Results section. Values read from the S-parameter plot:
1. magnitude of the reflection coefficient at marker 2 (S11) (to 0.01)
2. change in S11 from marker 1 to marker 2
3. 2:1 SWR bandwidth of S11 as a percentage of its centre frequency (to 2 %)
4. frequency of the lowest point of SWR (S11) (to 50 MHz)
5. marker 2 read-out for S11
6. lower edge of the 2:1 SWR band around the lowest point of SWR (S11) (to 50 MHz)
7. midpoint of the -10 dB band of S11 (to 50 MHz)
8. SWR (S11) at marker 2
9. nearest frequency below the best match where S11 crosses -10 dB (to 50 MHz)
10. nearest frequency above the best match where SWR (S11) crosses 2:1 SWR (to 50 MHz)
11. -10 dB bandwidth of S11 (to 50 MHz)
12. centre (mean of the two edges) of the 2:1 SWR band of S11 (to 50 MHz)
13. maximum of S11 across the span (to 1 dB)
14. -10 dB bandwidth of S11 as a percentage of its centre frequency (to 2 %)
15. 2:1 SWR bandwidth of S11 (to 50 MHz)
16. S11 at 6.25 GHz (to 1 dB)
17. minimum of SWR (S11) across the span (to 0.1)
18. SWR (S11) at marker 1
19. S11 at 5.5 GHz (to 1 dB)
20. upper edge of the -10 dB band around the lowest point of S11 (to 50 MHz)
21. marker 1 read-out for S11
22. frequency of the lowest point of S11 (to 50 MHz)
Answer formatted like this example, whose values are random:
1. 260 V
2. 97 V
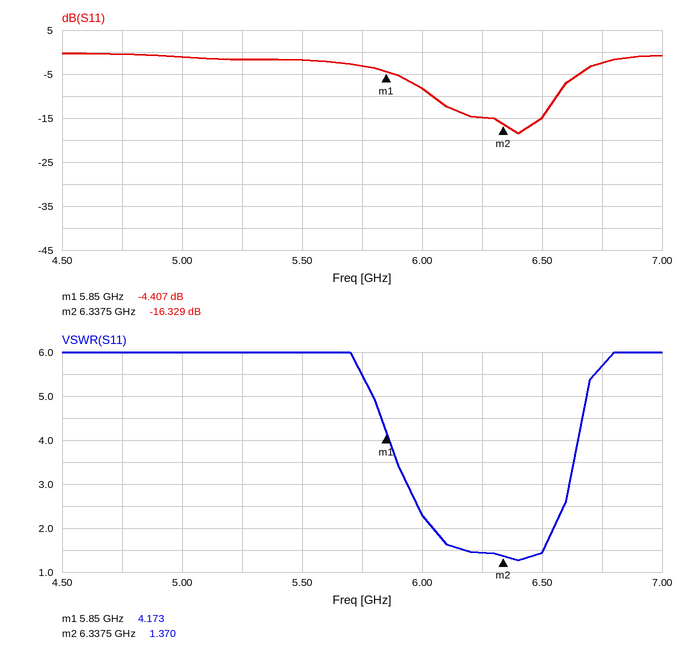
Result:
1. 0.15
2. -11.922 dB
3. 8 %
4. 6.40 GHz
5. -16.329 dB
6. 6.05 GHz
7. 6.30 GHz
8. 1.370
9. 6.05 GHz
10. 6.55 GHz
11. 500 MHz
12. 6.30 GHz
13. 0 dB
14. 8 %
15. 500 MHz
16. -15 dB
17. 1.3
18. 4.173
19. -2 dB
20. 6.55 GHz
21. -4.407 dB
22. 6.40 GHz
